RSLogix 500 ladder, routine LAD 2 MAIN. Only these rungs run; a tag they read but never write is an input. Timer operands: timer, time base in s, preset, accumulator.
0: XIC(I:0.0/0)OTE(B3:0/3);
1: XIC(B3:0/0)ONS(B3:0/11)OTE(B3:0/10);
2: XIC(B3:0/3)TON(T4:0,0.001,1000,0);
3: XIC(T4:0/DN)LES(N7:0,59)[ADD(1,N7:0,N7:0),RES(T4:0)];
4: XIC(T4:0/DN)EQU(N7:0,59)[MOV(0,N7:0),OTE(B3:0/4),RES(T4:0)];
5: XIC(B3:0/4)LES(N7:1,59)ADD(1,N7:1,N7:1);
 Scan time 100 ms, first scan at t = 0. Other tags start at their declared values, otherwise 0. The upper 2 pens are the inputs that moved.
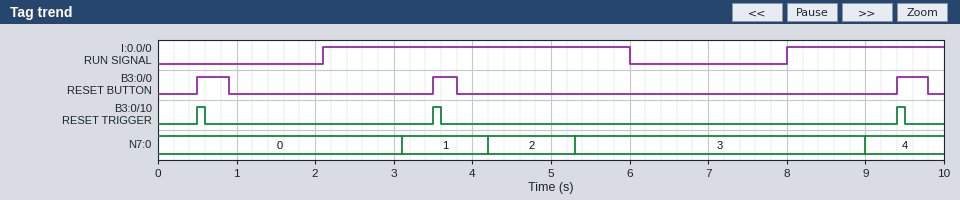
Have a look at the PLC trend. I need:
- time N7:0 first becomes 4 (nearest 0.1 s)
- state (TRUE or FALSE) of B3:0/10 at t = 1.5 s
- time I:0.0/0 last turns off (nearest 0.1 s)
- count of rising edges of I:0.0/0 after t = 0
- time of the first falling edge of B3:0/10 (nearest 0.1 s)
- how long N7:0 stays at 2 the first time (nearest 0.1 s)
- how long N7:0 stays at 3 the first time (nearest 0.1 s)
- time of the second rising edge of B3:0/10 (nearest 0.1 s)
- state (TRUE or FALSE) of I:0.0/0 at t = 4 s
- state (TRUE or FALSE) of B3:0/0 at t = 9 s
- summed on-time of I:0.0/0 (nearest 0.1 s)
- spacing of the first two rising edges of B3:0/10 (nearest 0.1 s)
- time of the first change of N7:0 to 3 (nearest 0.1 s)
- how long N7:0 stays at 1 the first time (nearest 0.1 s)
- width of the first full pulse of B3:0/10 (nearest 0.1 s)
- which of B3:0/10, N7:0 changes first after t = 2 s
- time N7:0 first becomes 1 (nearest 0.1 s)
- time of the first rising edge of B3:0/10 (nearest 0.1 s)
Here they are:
9.0 s
FALSE
6.0 s
2
0.6 s
1.1 s
3.7 s
3.5 s
TRUE
FALSE
5.9 s
3.0 s
5.3 s
1.1 s
0.1 s
N7:0
3.1 s
0.5 s
